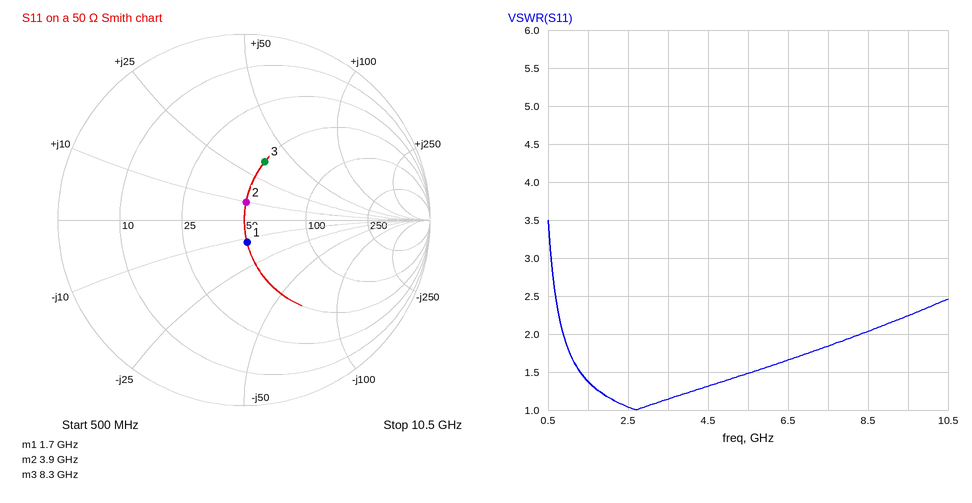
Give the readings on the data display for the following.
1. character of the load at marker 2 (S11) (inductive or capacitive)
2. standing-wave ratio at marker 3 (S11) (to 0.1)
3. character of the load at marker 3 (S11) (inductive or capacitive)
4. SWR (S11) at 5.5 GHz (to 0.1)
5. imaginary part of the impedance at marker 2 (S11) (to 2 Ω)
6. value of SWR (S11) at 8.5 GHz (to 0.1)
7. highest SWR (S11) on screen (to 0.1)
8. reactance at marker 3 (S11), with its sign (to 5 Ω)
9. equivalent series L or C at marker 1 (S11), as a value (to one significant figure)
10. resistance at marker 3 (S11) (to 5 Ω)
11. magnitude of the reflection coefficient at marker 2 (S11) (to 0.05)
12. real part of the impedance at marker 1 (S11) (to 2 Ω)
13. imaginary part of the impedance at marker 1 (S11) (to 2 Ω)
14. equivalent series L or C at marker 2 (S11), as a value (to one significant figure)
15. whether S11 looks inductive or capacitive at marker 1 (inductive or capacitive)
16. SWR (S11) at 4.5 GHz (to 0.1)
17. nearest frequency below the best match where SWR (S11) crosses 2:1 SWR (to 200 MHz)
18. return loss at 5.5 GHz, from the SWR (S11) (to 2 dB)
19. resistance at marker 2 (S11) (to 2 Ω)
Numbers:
inductive
2.0
inductive
1.5
+10 Ω
2.0
3.5
+35 Ω
8 pF
50 Ω
0.10
50 Ω
-12 Ω
400 pH
capacitive
1.3
800 MHz
14 dB
50 Ω
